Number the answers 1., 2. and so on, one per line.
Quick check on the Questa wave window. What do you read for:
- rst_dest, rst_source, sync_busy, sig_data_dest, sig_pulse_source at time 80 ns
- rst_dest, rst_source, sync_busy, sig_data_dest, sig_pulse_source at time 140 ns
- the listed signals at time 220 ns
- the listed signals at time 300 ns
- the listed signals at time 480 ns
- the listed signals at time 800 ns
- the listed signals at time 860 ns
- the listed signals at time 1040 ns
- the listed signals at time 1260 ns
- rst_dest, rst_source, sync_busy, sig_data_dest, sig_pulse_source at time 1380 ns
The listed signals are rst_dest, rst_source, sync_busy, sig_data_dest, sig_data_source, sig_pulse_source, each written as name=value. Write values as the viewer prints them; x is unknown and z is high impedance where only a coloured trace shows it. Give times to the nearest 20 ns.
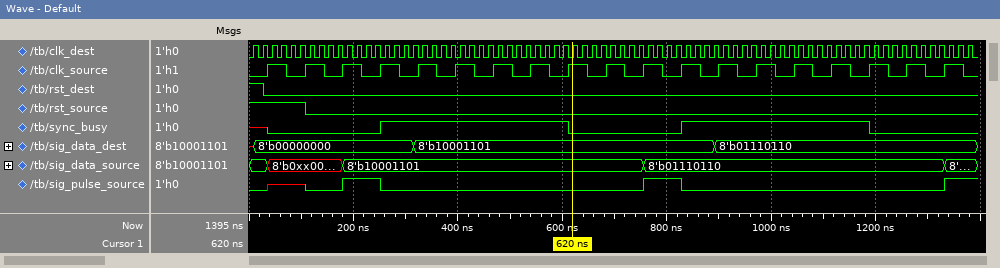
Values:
1. rst_dest=0, rst_source=1, sync_busy=0, sig_data_dest=8'b00000000, sig_pulse_source=x
2. rst_dest=0, rst_source=0, sync_busy=0, sig_data_dest=8'b00000000, sig_pulse_source=0
3. rst_dest=0, rst_source=0, sync_busy=0, sig_data_dest=8'b00000000, sig_data_source=8'b10001101, sig_pulse_source=1
4. rst_dest=0, rst_source=0, sync_busy=1, sig_data_dest=8'b00000000, sig_data_source=8'b10001101, sig_pulse_source=0
5. rst_dest=0, rst_source=0, sync_busy=1, sig_data_dest=8'b10001101, sig_data_source=8'b10001101, sig_pulse_source=0
6. rst_dest=0, rst_source=0, sync_busy=0, sig_data_dest=8'b10001101, sig_data_source=8'b01110110, sig_pulse_source=1
7. rst_dest=0, rst_source=0, sync_busy=1, sig_data_dest=8'b10001101, sig_data_source=8'b01110110, sig_pulse_source=0
8. rst_dest=0, rst_source=0, sync_busy=1, sig_data_dest=8'b01110110, sig_data_source=8'b01110110, sig_pulse_source=0
9. rst_dest=0, rst_source=0, sync_busy=0, sig_data_dest=8'b01110110, sig_data_source=8'b01110110, sig_pulse_source=0
10. rst_dest=0, rst_source=0, sync_busy=0, sig_data_dest=8'b01110110, sig_pulse_source=1
